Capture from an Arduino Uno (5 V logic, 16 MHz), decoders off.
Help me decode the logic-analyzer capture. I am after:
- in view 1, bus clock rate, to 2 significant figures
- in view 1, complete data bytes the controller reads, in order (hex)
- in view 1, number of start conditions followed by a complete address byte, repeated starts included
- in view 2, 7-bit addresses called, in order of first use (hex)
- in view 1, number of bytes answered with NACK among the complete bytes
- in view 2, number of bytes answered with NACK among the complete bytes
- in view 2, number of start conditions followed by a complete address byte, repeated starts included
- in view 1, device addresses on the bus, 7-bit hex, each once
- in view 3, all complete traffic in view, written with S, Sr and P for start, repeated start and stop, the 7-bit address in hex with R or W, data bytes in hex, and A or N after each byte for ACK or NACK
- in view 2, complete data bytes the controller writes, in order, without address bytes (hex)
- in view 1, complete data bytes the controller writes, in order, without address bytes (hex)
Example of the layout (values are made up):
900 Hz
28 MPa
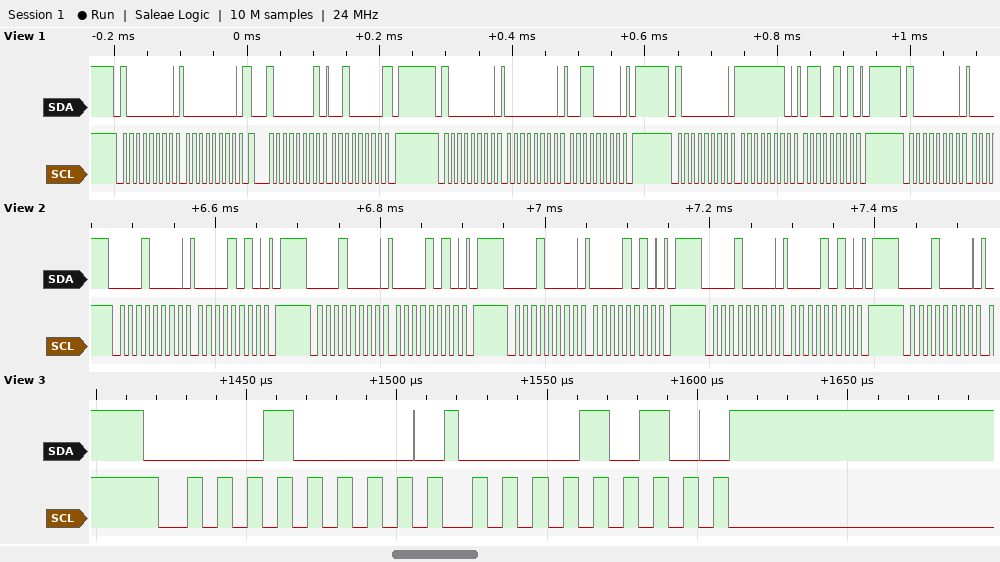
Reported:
100 kHz
20
5
0x08
1
0
5
0x40
S 08W A 0A A
0A 0A 0A 0A
00 00 30 FE 65
